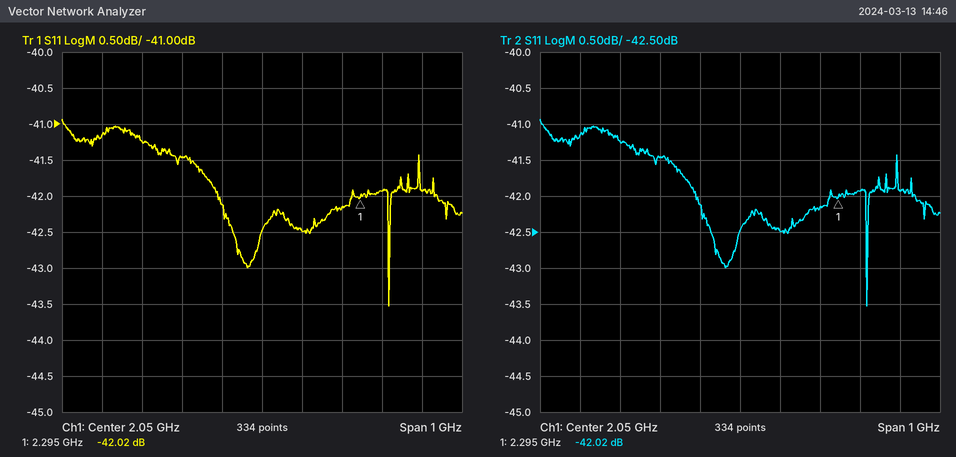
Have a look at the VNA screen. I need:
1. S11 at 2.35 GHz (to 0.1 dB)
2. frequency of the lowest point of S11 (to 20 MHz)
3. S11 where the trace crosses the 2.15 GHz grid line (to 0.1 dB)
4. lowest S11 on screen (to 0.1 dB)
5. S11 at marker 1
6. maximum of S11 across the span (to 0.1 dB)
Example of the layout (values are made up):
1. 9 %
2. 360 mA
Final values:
1. -41.9 dB
2. 2.36 GHz
3. -42.5 dB
4. -43.5 dB
5. -42.02 dB
6. -40.9 dB
